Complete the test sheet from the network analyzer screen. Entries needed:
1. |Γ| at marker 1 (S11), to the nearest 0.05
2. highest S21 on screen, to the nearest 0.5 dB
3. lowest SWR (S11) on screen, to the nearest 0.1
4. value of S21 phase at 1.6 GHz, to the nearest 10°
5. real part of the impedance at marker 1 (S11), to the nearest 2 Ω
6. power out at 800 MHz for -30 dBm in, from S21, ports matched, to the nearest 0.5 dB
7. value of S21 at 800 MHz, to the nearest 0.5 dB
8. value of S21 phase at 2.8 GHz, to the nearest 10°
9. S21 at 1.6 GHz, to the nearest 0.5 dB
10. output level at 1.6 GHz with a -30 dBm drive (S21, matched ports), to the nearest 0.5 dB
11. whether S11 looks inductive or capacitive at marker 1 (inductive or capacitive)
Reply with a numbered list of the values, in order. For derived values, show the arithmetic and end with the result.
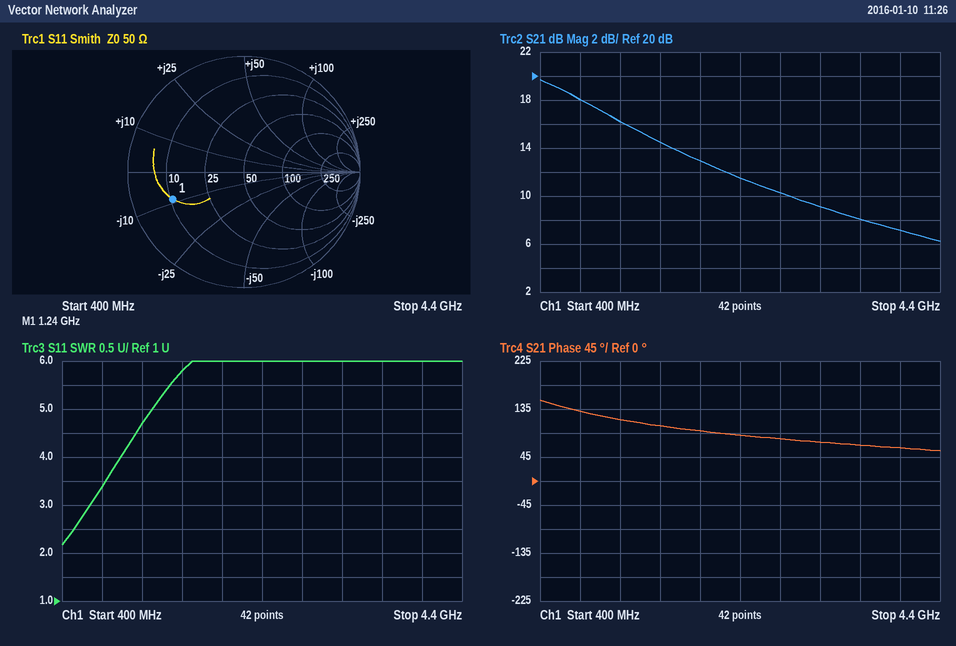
1. 0.65
2. 19.5 dB
3. 2.2
4. 100°
5. 10 Ω
6. -30 dBm + (18.0 dB) = -12.0 dBm
7. 18.0 dB
8. 80°
9. 14.5 dB
10. -30 dBm + (14.5 dB) = -15.5 dBm
11. capacitive
